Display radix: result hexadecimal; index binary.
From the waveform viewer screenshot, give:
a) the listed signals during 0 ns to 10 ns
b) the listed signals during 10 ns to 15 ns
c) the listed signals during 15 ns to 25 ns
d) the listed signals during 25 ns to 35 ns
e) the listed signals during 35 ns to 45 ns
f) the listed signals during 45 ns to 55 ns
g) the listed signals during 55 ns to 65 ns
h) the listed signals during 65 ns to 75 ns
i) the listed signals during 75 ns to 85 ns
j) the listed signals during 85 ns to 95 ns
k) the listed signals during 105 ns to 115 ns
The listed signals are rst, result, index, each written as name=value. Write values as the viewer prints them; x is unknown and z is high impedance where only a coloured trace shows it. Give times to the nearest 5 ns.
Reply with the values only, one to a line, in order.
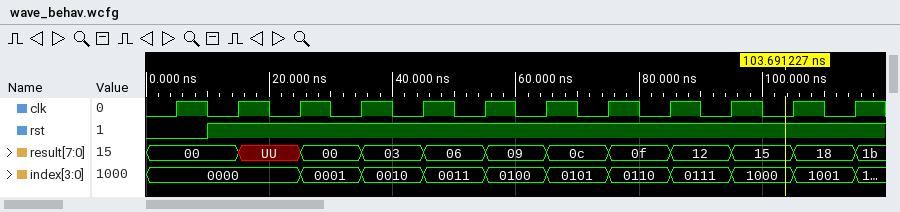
rst=0, result=00, index=0000
rst=1, result=00, index=0000
rst=1, result=UU, index=0000
rst=1, result=00, index=0001
rst=1, result=03, index=0010
rst=1, result=06, index=0011
rst=1, result=09, index=0100
rst=1, result=0c, index=0101
rst=1, result=0f, index=0110
rst=1, result=12, index=0111
rst=1, result=18, index=1001
